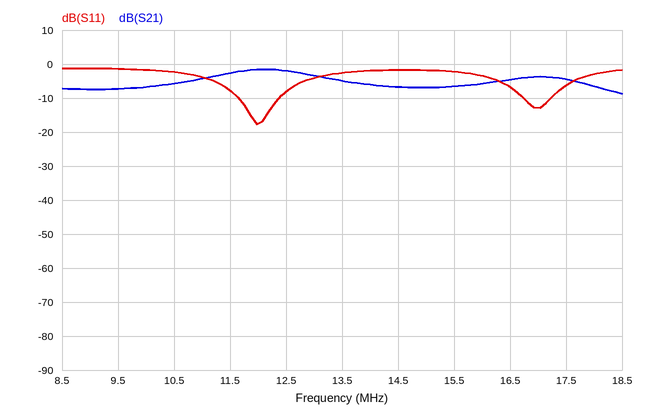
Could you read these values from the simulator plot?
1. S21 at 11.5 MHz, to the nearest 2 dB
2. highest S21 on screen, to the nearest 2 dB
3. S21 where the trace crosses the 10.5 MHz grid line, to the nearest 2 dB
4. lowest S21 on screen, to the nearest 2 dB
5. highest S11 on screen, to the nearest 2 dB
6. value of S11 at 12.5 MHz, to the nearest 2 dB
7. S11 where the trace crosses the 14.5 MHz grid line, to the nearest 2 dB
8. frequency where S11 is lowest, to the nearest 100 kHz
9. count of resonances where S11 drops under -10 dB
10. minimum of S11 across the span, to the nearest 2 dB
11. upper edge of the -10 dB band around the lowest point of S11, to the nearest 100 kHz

-2 dB
-2 dB
-6 dB
-8 dB
-2 dB
-8 dB
-2 dB
12.0 MHz
2
-18 dB
12.4 MHz
